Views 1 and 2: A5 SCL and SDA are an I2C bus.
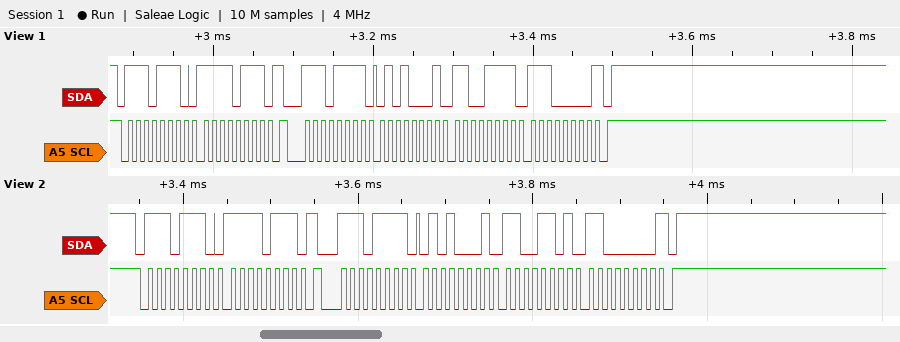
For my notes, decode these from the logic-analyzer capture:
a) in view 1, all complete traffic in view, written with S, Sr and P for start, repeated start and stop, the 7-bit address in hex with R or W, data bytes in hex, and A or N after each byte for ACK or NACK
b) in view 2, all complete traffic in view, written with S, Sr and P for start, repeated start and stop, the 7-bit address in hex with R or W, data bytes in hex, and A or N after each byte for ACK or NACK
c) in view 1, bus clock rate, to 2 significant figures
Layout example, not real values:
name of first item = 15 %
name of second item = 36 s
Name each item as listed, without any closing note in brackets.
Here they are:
in view 1, all complete traffic in view, written with S, Sr and P for start, repeated start and stop, the 7-bit address in hex with R or W, data bytes in hex, and A or N after each byte for ACK or NACK = S 77W A F7 A Sr 77R A 51 A CF A E0 N P
in view 2, all complete traffic in view, written with S, Sr and P for start, repeated start and stop, the 7-bit address in hex with R or W, data bytes in hex, and A or N after each byte for ACK or NACK = S 77W A F7 A Sr 77R A 51 A CD A C0 N P
in view 1, bus clock rate, to 2 significant figures = 100 kHz
